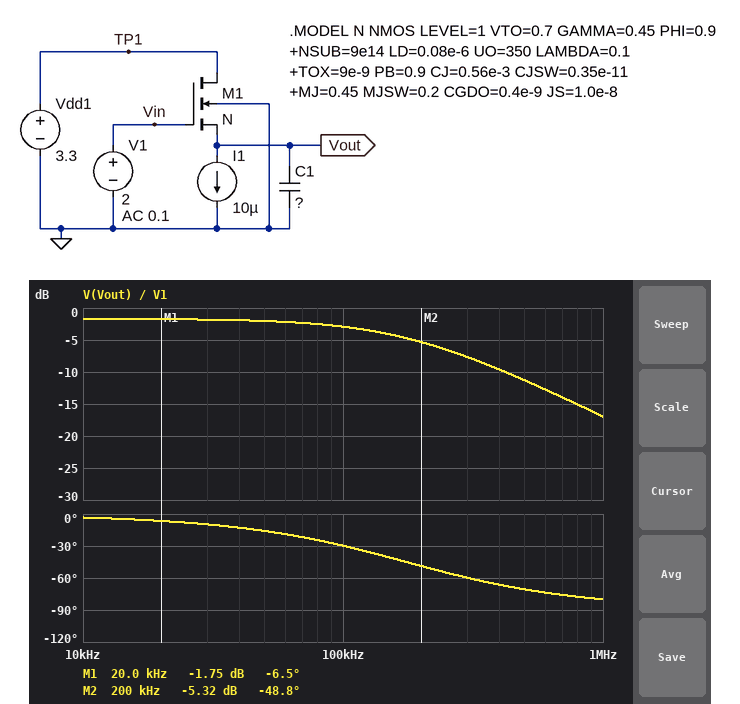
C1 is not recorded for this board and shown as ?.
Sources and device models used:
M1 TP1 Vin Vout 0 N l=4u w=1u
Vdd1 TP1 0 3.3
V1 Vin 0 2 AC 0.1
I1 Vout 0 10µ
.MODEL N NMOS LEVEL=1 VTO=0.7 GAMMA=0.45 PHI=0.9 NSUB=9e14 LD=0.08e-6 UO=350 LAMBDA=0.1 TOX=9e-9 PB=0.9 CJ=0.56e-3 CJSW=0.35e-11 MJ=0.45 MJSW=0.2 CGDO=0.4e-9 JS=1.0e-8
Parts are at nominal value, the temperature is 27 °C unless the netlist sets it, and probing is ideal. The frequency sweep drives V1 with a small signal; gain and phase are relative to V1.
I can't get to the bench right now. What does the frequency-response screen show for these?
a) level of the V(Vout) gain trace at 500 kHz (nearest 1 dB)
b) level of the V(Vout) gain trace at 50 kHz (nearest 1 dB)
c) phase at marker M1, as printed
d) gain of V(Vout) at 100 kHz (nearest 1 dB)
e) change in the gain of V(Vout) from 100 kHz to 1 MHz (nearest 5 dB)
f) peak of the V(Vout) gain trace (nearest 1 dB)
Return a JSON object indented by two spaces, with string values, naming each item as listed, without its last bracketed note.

{
  "level of the V(Vout) gain trace at 500 kHz": "-11 dB",
  "level of the V(Vout) gain trace at 50 kHz": "-2 dB",
  "phase at marker M1, as printed": "-6.5 deg",
  "gain of V(Vout) at 100 kHz": "-3 dB",
  "change in the gain of V(Vout) from 100 kHz to 1 MHz": "-15 dB",
  "peak of the V(Vout) gain trace": "-2 dB"
}
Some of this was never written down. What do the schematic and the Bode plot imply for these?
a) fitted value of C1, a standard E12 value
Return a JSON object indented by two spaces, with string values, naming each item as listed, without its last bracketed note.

{
  "fitted value of C1, a standard E12 value": "33 pF"
}
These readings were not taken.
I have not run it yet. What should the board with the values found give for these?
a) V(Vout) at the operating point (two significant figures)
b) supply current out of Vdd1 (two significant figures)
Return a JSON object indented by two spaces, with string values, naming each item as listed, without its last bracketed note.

{
  "V(Vout) at the operating point": "520 mV",
  "supply current out of Vdd1": "10 µA"
}
